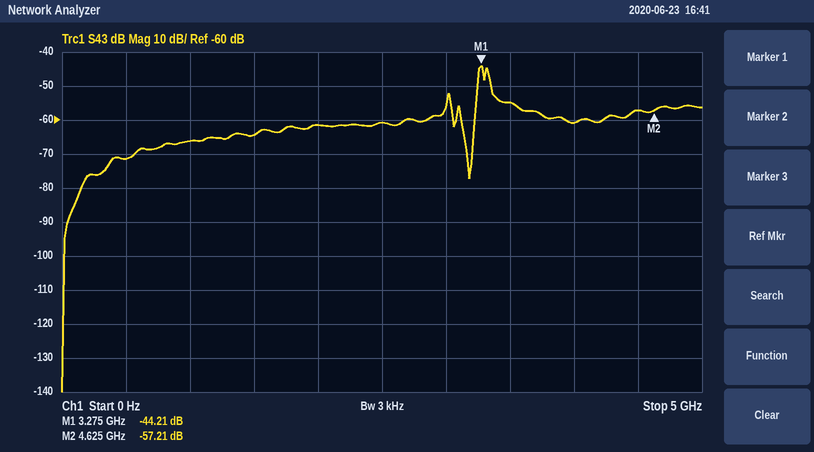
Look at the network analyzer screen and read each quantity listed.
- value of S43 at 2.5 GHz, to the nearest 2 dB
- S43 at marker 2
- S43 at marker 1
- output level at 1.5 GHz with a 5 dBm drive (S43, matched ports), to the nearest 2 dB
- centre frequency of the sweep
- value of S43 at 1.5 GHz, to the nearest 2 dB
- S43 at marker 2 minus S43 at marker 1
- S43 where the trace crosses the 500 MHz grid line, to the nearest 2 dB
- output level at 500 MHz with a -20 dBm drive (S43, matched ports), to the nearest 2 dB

-60 dB
-57.21 dB
-44.21 dB
-60 dBm
2.5 GHz
-64 dB
-13.00 dB
-72 dB
-92 dBm
